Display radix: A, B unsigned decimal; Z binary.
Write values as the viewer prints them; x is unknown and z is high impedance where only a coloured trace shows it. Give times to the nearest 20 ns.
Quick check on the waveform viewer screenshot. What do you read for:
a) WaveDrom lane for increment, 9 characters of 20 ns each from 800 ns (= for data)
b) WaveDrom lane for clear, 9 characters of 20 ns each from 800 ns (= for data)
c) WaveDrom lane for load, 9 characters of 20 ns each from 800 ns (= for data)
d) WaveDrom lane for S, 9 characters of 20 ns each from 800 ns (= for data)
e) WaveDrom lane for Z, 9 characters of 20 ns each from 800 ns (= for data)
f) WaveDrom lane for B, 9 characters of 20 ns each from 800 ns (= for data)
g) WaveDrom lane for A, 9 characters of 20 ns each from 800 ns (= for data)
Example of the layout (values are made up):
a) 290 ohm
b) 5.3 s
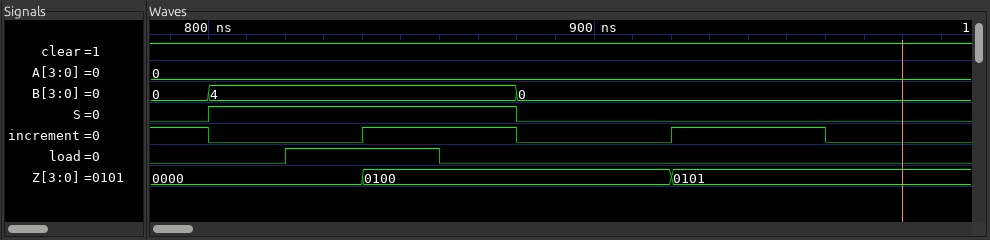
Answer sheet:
a) {name: 'increment', wave: '0.1.0.1.0'}
b) {name: 'clear', wave: '1........'}
c) {name: 'load', wave: '01.0.....'}
d) {name: 'S', wave: '1...0....'}
e) {name: 'Z', wave: '=.=...=..', data: '0000 0100 0101'}
f) {name: 'B', wave: '=...=....', data: '4 0'}
g) {name: 'A', wave: '=........', data: '0'}
